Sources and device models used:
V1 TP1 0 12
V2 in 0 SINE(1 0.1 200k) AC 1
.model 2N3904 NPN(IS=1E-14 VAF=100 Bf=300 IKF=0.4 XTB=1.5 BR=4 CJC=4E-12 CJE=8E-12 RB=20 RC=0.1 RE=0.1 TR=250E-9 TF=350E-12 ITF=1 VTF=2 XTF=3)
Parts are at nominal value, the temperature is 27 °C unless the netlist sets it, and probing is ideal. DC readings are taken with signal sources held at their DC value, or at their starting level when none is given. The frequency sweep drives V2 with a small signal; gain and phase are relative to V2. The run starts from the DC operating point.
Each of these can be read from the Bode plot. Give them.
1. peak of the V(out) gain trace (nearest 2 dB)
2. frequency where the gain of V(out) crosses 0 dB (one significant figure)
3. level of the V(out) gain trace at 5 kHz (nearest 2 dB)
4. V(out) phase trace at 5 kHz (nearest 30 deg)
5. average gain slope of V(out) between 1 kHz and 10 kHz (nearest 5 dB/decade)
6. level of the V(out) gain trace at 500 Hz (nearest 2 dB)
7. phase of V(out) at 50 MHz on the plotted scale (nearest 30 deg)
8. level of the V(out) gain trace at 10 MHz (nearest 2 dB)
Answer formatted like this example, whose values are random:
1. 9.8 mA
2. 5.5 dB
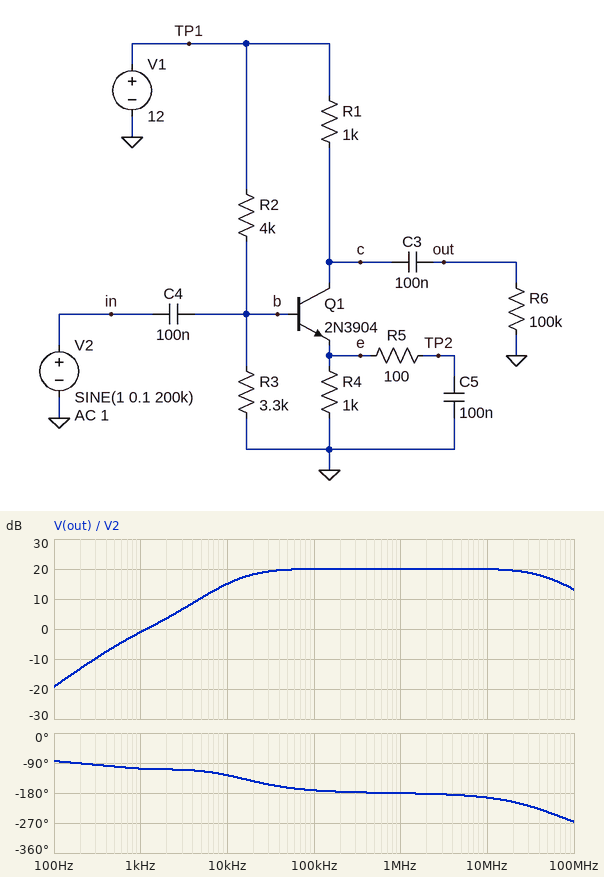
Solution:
1. 20 dB
2. 1 kHz
3. 10 dB
4. -120 deg
5. 15 dB/decade
6. -6 dB
7. -240 deg
8. 20 dB
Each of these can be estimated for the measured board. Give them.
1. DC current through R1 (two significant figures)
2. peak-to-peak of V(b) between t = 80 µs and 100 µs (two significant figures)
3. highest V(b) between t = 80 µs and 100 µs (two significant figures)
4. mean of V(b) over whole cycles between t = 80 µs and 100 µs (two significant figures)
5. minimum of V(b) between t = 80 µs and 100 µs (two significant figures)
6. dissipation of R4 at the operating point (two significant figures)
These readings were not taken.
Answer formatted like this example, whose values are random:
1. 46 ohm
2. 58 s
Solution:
1. 4.7 mA
2. 200 mV
3. 5.5 V
4. 5.4 V
5. 5.3 V
6. 22 mW
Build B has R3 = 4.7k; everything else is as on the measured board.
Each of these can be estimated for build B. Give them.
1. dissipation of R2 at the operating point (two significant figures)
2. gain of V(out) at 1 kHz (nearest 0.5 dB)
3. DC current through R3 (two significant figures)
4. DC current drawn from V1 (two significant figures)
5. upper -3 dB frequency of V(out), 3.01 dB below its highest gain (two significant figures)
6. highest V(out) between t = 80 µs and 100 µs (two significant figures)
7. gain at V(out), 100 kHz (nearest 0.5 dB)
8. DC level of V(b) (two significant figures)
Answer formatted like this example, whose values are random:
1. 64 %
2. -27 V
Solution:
1. 7.7 mW
2. -0.5 dB
3. 1.4 mA
4. 7.1 mA
5. 30 MHz
6. 1.1 V
7. 20.0 dB
8. 6.4 V
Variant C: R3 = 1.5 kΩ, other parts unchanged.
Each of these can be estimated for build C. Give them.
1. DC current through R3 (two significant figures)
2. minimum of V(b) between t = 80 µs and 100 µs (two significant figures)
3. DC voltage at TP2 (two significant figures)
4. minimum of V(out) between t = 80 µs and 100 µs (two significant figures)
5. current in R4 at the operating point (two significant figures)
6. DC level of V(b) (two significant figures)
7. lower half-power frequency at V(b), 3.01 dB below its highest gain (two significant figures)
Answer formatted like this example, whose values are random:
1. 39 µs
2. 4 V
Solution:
1. 2.2 mA
2. 3.2 V
3. 2.6 V
4. -980 mV
5. 2.6 mA
6. 3.3 V
7. 1.5 kHz
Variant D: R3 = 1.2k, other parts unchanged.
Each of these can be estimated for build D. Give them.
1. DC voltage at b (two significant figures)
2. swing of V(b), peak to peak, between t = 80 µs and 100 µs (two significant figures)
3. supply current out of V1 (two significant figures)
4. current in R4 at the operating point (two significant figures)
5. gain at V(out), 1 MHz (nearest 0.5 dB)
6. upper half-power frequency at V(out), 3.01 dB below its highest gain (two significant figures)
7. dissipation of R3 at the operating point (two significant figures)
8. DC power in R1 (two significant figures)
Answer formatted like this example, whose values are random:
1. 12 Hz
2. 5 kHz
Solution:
1. 2.8 V
2. 200 mV
3. 4.4 mA
4. 2.1 mA
5. 19.5 dB
6. 69 MHz
7. 6.4 mW
8. 4.3 mW
